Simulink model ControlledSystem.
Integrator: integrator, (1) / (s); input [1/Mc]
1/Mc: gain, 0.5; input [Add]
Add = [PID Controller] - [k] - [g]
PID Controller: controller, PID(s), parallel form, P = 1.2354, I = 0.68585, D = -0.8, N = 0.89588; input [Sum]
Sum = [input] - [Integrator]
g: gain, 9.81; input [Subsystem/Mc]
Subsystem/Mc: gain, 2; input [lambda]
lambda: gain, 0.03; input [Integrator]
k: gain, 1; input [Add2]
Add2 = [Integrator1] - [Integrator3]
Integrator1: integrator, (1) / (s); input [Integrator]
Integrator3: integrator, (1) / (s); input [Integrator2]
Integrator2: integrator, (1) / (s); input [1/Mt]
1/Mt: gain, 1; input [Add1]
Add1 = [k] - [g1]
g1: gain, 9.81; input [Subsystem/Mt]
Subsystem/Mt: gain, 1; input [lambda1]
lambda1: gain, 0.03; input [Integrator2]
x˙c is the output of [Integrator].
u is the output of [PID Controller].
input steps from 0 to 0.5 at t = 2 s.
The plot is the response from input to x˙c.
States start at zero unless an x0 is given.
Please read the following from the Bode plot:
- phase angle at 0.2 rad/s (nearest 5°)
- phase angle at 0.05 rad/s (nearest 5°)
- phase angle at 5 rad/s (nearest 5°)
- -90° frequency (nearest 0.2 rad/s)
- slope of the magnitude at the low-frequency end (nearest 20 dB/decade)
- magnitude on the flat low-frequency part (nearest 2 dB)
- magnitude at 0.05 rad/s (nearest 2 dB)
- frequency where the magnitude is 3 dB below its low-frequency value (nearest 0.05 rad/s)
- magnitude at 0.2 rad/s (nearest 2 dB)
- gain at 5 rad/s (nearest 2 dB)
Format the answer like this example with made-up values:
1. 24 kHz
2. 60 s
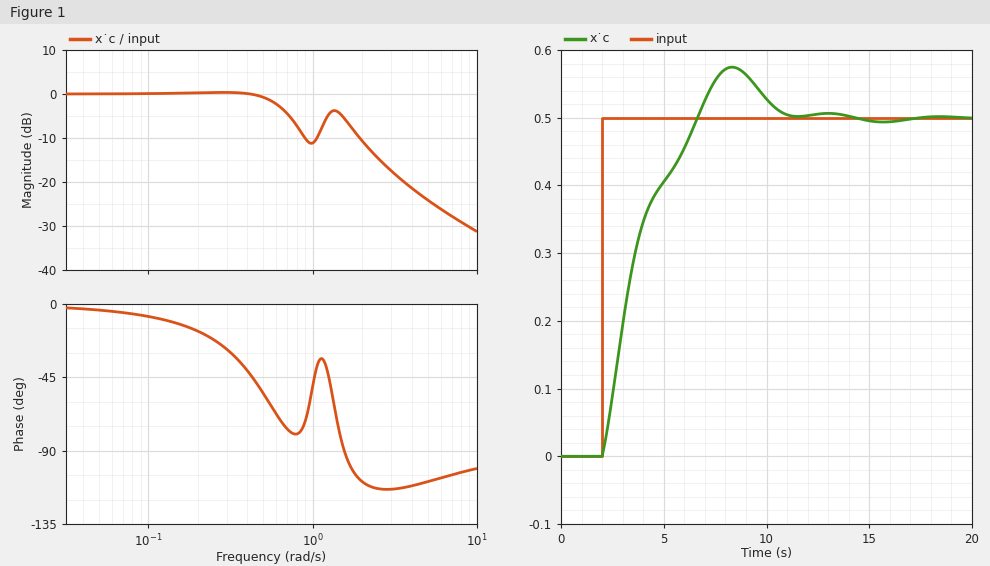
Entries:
1. -15°
2. -5°
3. -110°
4. 1.6 rad/s
5. 0 dB/decade
6. 0 dB
7. 0 dB
8. 0.65 rad/s
9. 0 dB
10. -24 dB
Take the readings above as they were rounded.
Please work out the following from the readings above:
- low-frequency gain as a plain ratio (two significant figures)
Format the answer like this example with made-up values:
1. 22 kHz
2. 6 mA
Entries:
1. 1.0
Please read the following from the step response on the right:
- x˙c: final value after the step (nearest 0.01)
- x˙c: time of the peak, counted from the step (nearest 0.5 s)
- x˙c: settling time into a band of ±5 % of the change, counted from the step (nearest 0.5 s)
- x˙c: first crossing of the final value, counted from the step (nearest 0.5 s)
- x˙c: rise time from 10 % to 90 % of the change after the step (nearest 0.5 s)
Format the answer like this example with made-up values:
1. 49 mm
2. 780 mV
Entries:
1. 0.50
2. 6.5 s
3. 8.0 s
4. 4.5 s
5. 3.5 s
